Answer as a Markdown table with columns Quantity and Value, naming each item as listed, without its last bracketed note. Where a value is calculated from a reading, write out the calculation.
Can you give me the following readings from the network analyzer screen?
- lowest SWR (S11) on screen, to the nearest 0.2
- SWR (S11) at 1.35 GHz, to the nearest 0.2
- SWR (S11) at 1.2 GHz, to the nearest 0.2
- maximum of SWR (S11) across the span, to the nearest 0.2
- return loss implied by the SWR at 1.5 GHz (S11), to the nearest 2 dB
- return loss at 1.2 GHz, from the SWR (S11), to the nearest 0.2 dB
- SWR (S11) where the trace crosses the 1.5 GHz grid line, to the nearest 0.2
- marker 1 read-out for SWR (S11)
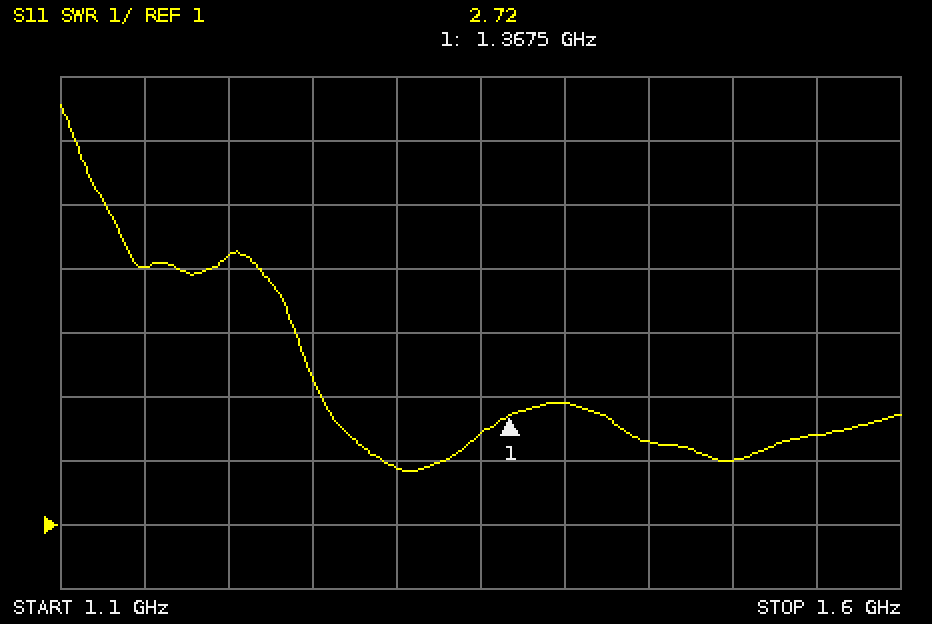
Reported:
| Quantity | Value |
|---|---|
| lowest SWR (S11) on screen, to the nearest 0.2 | 1.8 |
| SWR (S11) at 1.35 GHz, to the nearest 0.2 | 2.4 |
| SWR (S11) at 1.2 GHz, to the nearest 0.2 | 5.2 |
| maximum of SWR (S11) across the span, to the nearest 0.2 | 7.6 |
| return loss implied by the SWR at 1.5 GHz (S11), to the nearest 2 dB | −20 log10((2 − 1)/(2 + 1)) ≈ 10 dB |
| return loss at 1.2 GHz, from the SWR (S11), to the nearest 0.2 dB | −20 log10((5.2 − 1)/(5.2 + 1)) ≈ 3.4 dB |
| SWR (S11) where the trace crosses the 1.5 GHz grid line, to the nearest 0.2 | 2.0 |
| marker 1 read-out for SWR | 2.72 |
